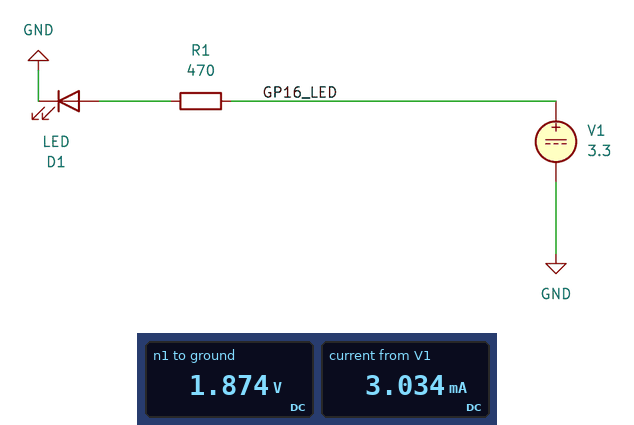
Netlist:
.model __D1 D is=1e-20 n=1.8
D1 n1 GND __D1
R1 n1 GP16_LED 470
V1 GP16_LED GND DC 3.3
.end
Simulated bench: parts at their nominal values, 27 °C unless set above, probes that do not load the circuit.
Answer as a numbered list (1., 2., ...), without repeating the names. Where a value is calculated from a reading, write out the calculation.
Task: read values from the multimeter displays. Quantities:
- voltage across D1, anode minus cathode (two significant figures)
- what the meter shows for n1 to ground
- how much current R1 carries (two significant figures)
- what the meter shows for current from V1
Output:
1. 1.874 V = 1.9 V
2. 1.874 V
3. (3.3 V - 1.874 V) / 470 Ω = 3.0 mA
4. 3.034 mA
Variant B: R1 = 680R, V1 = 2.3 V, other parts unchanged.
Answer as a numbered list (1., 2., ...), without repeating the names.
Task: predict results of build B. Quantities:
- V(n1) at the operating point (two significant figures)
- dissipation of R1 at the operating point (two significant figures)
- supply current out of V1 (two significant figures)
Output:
1. 1.8 V
2. 360 µW
3. 720 µA
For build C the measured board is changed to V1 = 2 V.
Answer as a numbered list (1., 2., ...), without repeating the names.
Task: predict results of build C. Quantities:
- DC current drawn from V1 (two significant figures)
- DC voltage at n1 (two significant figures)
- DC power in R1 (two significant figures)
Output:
1. 460 µA
2. 1.8 V
3. 98 µW
